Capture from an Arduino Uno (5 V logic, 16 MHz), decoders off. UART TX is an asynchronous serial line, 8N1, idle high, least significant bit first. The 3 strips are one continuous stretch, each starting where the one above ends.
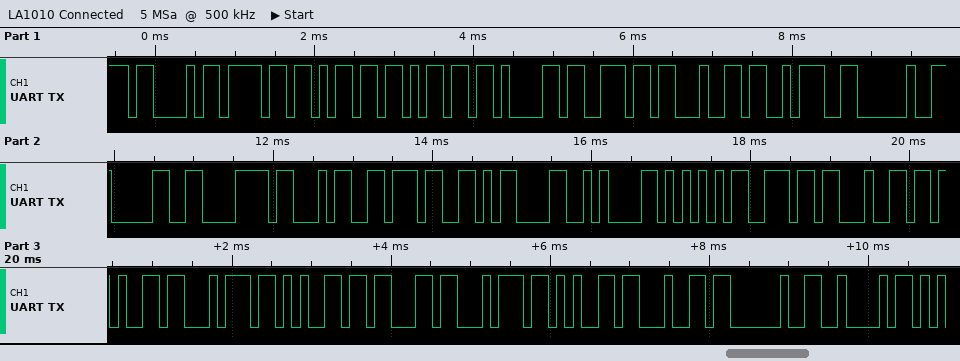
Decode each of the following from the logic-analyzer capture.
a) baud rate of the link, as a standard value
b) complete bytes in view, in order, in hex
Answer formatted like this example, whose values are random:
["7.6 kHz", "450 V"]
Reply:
["9600 baud", "43 6F 6D 6D 61 6E 64 3A 20 30 78 34 37 0D 0A 55 6E 64 65 74 65 63 74 65 64 20 42"]
